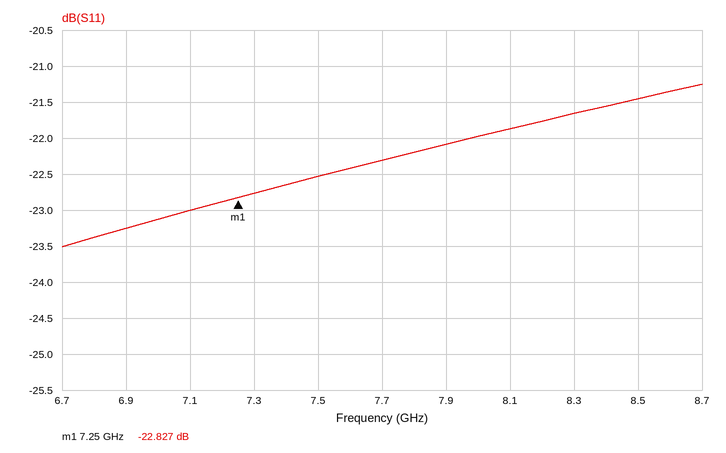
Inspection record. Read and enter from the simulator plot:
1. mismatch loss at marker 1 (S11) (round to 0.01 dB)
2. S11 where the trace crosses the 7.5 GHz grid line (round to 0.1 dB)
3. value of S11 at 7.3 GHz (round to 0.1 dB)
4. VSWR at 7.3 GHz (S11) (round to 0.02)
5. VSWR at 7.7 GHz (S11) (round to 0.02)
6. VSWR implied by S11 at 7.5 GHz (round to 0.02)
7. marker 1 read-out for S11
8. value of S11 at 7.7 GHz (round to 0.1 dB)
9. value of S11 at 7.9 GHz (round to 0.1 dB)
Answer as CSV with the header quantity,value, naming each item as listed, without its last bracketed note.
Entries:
quantity,value
mismatch loss at marker 1 (S11),0.02 dB
S11 where the trace crosses the 7.5 GHz grid line,-22.5 dB
value of S11 at 7.3 GHz,-22.8 dB
VSWR at 7.3 GHz (S11),1.16
VSWR at 7.7 GHz (S11),1.16
VSWR implied by S11 at 7.5 GHz,1.16
marker 1 read-out for S11,-22.827 dB
value of S11 at 7.7 GHz,-22.3 dB
value of S11 at 7.9 GHz,-22.1 dB
